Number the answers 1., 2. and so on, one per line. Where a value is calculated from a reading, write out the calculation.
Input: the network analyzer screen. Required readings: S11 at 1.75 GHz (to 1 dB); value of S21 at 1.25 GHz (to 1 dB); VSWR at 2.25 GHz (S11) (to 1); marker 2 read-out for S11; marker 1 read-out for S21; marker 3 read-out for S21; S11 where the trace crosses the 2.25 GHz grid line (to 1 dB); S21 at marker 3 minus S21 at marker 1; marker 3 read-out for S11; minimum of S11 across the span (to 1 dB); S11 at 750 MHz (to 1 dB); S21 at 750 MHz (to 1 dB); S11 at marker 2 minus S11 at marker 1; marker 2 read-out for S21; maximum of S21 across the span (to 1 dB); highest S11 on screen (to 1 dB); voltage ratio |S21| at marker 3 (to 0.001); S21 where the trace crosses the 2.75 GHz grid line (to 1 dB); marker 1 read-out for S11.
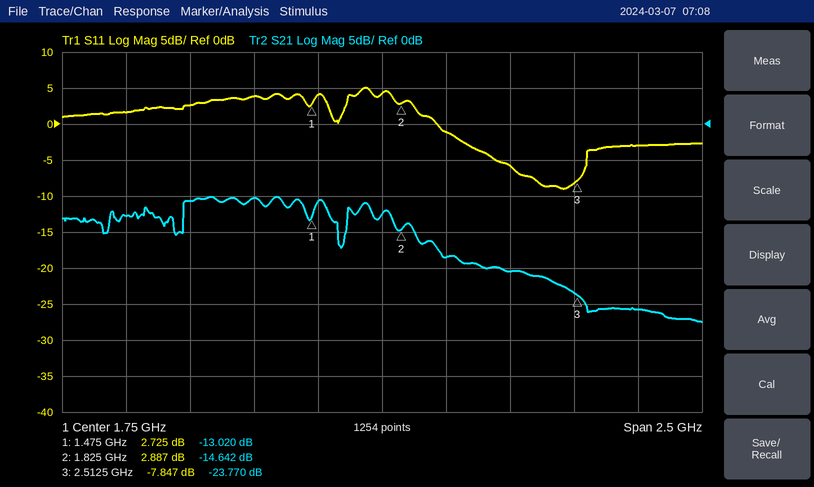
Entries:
1. 4 dB
2. -10 dB
3. |Γ| = 10^(-6/20) = 0.5012; VSWR = (1 + 0.5012)/(1 − 0.5012) ≈ 3
4. 2.887 dB
5. -13.020 dB
6. -23.770 dB
7. -6 dB
8. -23.77 − (-13.02) = -10.750 dB
9. -7.847 dB
10. -9 dB
11. 2 dB
12. -13 dB
13. 2.887 − (2.725) = 0.162 dB
14. -14.642 dB
15. -10 dB
16. 5 dB
17. 10^(-23.77/20) ≈ 0.065
18. -26 dB
19. 2.725 dB
